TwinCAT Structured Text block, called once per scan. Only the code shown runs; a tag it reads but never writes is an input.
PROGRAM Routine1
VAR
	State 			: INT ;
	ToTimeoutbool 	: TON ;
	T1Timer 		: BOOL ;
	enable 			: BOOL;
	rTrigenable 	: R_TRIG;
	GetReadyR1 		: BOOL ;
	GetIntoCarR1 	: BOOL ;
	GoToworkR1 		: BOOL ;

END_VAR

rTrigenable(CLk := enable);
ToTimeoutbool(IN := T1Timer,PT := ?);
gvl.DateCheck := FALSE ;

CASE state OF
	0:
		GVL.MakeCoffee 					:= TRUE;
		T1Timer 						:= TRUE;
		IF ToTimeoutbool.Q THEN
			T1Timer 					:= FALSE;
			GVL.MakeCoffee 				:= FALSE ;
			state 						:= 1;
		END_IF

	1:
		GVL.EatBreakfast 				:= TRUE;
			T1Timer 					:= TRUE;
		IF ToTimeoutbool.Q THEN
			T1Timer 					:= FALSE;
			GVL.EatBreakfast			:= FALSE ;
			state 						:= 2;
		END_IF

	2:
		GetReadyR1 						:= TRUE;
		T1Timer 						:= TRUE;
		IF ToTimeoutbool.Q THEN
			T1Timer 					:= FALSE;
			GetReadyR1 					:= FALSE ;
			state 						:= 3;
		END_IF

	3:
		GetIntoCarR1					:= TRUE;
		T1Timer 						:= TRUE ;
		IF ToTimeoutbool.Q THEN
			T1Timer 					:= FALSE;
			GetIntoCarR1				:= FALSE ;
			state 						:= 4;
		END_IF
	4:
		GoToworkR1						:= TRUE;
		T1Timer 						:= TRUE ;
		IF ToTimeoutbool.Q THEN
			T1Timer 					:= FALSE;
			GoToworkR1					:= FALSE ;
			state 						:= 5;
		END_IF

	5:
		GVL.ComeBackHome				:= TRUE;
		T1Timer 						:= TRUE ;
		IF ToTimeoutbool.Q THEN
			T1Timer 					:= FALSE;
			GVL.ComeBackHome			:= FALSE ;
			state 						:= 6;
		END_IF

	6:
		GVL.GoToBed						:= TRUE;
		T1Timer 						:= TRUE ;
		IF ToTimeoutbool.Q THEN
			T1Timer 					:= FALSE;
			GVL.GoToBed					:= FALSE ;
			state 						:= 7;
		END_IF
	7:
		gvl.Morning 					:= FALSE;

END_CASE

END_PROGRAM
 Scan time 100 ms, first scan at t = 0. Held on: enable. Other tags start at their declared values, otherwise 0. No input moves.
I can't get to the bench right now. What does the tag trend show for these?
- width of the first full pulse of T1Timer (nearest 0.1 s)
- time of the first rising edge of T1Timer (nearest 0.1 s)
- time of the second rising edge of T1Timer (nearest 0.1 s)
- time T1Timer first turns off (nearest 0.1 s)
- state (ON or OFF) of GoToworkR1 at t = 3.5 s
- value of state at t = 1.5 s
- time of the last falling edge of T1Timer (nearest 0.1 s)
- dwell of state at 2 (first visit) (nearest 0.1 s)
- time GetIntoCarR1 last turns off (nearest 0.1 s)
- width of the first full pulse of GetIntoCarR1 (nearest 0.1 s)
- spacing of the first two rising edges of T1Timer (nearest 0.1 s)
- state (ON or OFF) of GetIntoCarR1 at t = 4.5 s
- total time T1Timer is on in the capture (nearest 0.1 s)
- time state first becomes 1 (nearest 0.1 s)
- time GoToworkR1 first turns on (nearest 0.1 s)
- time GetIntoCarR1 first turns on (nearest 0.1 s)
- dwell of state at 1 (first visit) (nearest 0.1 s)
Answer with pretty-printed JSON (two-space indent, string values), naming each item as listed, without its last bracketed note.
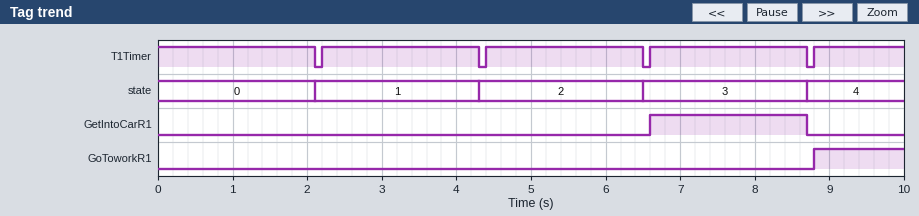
{
  "width of the first full pulse of T1Timer": "2.1 s",
  "time of the first rising edge of T1Timer": "2.2 s",
  "time of the second rising edge of T1Timer": "4.4 s",
  "time T1Timer first turns off": "2.1 s",
  "state (ON or OFF) of GoToworkR1 at t = 3.5 s": "OFF",
  "value of state at t = 1.5 s": "0",
  "time of the last falling edge of T1Timer": "8.7 s",
  "dwell of state at 2 (first visit)": "2.2 s",
  "time GetIntoCarR1 last turns off": "8.7 s",
  "width of the first full pulse of GetIntoCarR1": "2.1 s",
  "spacing of the first two rising edges of T1Timer": "2.2 s",
  "state (ON or OFF) of GetIntoCarR1 at t = 4.5 s": "OFF",
  "total time T1Timer is on in the capture": "9.6 s",
  "time state first becomes 1": "2.1 s",
  "time GoToworkR1 first turns on": "8.8 s",
  "time GetIntoCarR1 first turns on": "6.6 s",
  "dwell of state at 1 (first visit)": "2.2 s"
}
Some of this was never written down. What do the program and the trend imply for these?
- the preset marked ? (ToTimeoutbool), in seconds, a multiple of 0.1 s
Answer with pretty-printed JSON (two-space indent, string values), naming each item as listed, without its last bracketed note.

{
  "the preset marked ? (ToTimeoutbool), in seconds, a multiple of 0.1 s": "2.0 s"
}
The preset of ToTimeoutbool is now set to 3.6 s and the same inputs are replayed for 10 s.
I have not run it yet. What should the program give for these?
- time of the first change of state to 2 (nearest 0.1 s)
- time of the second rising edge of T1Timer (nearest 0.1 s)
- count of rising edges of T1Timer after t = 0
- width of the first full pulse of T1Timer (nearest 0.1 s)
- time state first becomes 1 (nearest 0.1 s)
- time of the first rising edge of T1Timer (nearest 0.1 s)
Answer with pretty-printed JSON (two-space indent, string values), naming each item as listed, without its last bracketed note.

{
  "time of the first change of state to 2": "7.5 s",
  "time of the second rising edge of T1Timer": "7.6 s",
  "count of rising edges of T1Timer after t = 0": "2",
  "width of the first full pulse of T1Timer": "3.7 s",
  "time state first becomes 1": "3.7 s",
  "time of the first rising edge of T1Timer": "3.8 s"
}
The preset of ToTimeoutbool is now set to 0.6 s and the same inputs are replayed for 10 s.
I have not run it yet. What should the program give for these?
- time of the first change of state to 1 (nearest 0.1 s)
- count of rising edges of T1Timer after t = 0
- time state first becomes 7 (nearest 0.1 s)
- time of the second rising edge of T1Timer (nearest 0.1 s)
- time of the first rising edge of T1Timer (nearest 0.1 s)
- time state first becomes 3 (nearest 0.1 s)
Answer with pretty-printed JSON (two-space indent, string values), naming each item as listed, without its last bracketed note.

{
  "time of the first change of state to 1": "0.7 s",
  "count of rising edges of T1Timer after t = 0": "6",
  "time state first becomes 7": "5.5 s",
  "time of the second rising edge of T1Timer": "1.6 s",
  "time of the first rising edge of T1Timer": "0.8 s",
  "time state first becomes 3": "2.3 s"
}
